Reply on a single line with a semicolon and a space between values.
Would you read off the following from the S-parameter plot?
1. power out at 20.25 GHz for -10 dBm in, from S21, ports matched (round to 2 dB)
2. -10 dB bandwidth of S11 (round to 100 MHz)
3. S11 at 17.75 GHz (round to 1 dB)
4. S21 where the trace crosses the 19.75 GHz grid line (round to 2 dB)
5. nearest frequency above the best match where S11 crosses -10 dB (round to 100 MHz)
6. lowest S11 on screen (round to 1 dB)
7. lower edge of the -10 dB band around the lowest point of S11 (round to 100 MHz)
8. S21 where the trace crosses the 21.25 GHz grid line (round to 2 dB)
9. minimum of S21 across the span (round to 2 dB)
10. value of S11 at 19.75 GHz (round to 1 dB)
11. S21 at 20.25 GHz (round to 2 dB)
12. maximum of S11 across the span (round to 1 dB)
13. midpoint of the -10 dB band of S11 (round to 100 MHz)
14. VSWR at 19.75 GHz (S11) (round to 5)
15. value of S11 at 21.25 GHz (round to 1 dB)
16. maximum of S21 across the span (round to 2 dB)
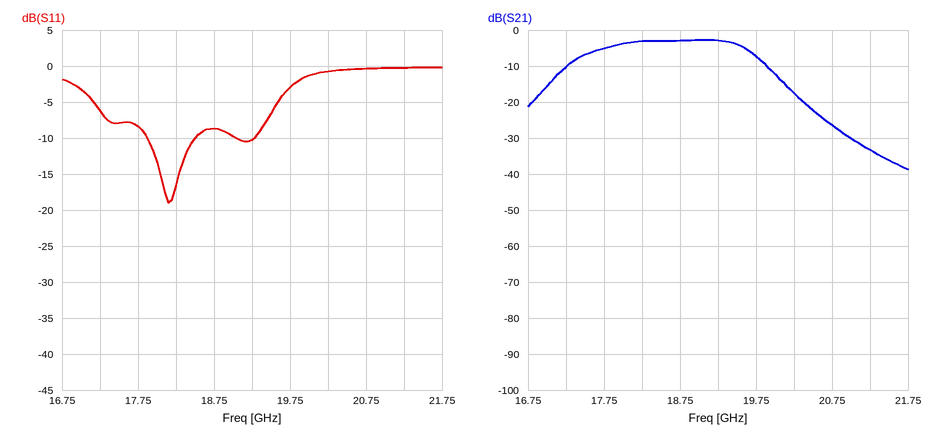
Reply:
-28 dBm; 600 MHz; -8 dB; -8 dB; 18.5 GHz; -19 dB; 17.9 GHz; -34 dB; -38 dB; -3 dB; -18 dB; 0 dB; 18.2 GHz; 5; 0 dB; -2 dB
